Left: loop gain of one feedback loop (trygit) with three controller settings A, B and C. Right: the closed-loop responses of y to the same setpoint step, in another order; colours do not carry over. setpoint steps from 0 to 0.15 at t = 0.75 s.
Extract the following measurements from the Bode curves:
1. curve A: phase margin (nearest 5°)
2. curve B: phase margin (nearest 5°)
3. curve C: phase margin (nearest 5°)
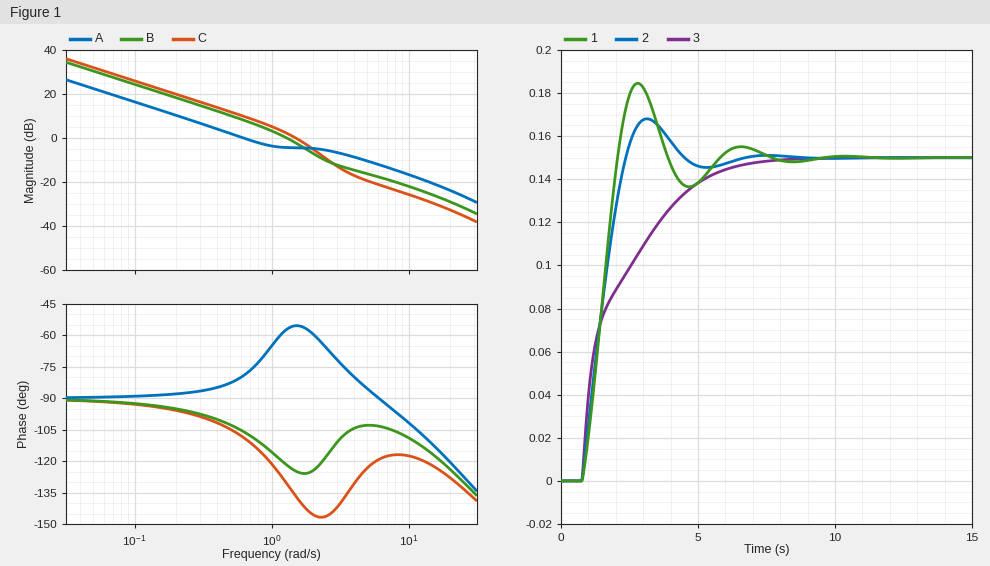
100°
60°
45°
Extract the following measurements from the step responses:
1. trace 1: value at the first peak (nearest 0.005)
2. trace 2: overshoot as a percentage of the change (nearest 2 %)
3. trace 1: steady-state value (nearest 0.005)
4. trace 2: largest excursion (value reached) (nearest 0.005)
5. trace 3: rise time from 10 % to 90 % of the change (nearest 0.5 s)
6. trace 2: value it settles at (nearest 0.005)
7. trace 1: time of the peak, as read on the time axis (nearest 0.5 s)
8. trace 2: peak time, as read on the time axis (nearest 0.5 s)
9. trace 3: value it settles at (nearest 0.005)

0.185
12 %
0.150
0.170
4.0 s
0.150
3.0 s
3.0 s
0.150
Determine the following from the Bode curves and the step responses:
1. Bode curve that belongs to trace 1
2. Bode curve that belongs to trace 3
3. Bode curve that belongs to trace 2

C
A
B
